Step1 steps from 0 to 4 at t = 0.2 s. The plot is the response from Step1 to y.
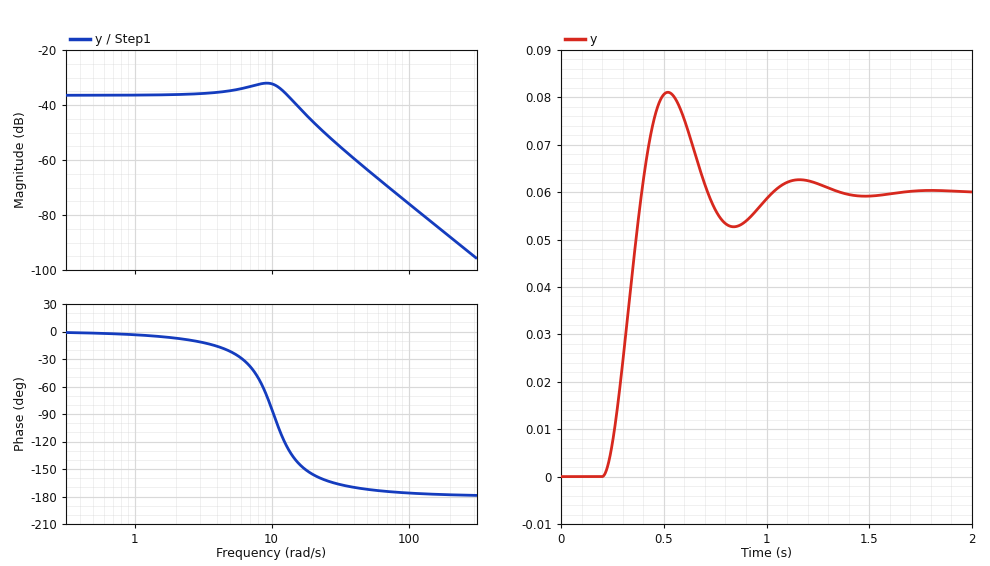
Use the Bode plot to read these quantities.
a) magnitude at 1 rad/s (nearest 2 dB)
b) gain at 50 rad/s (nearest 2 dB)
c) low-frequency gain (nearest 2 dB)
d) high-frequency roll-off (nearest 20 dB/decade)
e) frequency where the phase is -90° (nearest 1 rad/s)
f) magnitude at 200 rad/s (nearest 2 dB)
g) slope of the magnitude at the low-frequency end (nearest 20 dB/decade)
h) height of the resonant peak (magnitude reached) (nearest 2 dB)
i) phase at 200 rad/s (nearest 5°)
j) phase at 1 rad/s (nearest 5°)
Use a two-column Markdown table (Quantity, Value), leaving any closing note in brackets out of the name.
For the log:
| Quantity | Value |
|---|---|
| magnitude at 1 rad/s | -36 dB |
| gain at 50 rad/s | -64 dB |
| low-frequency gain | -36 dB |
| high-frequency roll-off | -40 dB/decade |
| frequency where the phase is -90° | 10 rad/s |
| magnitude at 200 rad/s | -88 dB |
| slope of the magnitude at the low-frequency end | 0 dB/decade |
| height of the resonant peak (magnitude reached) | -32 dB |
| phase at 200 rad/s | -180° |
| phase at 1 rad/s | -5° |
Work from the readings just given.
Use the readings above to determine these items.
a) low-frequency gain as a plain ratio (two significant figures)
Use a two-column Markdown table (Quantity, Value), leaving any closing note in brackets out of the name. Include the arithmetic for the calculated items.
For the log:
| Quantity | Value |
|---|---|
| low-frequency gain as a plain ratio | 10^(-36 / 20) = 0.016 |
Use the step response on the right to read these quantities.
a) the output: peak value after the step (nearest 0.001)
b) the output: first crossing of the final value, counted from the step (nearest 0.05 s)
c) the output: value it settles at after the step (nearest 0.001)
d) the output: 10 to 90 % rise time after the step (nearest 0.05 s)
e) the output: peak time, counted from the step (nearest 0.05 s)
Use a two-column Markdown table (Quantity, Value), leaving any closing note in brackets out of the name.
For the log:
| Quantity | Value |
|---|---|
| the output: peak value after the step | 0.081 |
| the output: first crossing of the final value, counted from the step | 0.20 s |
| the output: value it settles at after the step | 0.060 |
| the output: 10 to 90 % rise time after the step | 0.15 s |
| the output: peak time, counted from the step | 0.30 s |
